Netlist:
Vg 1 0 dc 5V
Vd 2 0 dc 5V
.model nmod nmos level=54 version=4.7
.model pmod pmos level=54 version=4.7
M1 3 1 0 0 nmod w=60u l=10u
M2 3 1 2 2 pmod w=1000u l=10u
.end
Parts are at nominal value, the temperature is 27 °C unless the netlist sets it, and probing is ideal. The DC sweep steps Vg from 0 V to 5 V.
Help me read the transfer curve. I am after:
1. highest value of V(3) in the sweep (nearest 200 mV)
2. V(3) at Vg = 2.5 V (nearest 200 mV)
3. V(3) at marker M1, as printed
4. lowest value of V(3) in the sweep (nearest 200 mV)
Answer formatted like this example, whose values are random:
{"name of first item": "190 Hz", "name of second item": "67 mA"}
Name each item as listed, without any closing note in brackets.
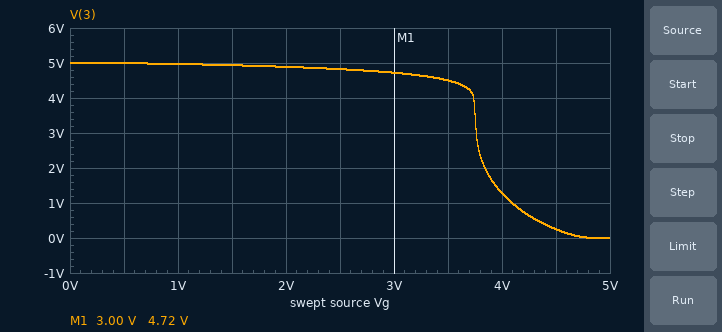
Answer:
{"highest value of V(3) in the sweep": "5.0 V", "V(3) at Vg = 2.5 V": "4.8 V", "V(3) at marker M1, as printed": "4.72 V", "lowest value of V(3) in the sweep": "0 V"}
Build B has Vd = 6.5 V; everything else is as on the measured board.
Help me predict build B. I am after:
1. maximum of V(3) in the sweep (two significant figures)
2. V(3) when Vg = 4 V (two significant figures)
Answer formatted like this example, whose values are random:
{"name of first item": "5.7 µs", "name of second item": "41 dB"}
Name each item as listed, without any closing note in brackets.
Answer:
{"maximum of V(3) in the sweep": "6.5 V", "V(3) when Vg = 4 V": "6.1 V"}
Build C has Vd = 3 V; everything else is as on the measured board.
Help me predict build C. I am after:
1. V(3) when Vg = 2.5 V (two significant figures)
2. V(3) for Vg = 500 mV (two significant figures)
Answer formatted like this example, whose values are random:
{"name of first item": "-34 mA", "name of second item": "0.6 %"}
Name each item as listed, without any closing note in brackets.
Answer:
{"V(3) when Vg = 2.5 V": "280 mV", "V(3) for Vg = 500 mV": "3.0 V"}
